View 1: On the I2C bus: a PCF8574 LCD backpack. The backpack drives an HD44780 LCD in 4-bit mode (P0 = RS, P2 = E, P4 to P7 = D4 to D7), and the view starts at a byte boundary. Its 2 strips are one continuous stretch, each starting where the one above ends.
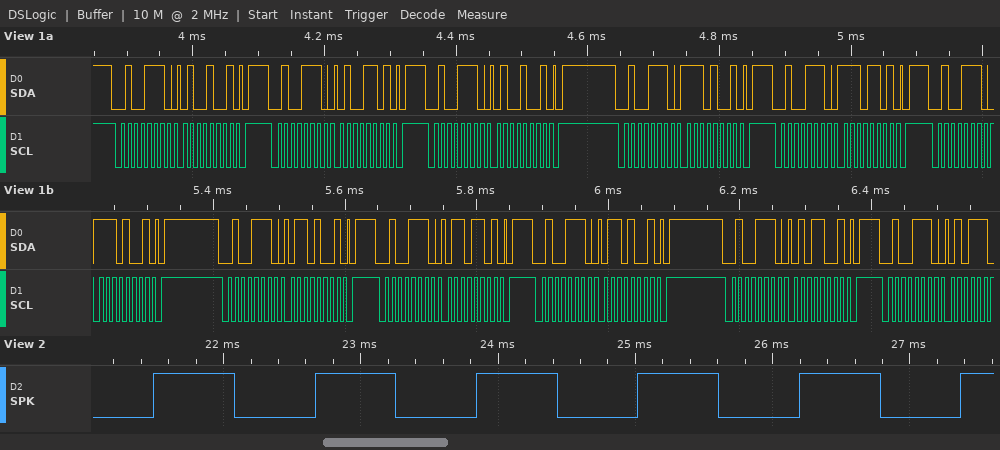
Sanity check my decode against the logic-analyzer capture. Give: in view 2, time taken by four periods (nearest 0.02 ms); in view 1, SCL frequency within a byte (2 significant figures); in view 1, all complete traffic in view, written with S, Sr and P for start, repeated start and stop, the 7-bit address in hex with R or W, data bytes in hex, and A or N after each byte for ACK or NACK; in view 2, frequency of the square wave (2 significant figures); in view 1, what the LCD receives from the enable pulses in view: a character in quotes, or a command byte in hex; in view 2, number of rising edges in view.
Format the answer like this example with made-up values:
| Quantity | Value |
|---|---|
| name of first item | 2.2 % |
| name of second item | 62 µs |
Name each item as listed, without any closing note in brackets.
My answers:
| Quantity | Value |
|---|---|
| in view 2, time taken by four periods | 4.70 ms |
| in view 1, SCL frequency within a byte | 100 kHz |
| in view 1, all complete traffic in view, written with S, Sr and P for start, repeated start and stop, the 7-bit address in hex with R or W, data bytes in hex, and A or N after each byte for ACK or NACK | S 27W A 49 A P S 27W A 4D A P S 27W A 49 A P S 27W A E9 A P S 27W A ED A P S 27W A E9 A P S 27W A 69 A P S 27W A 6D A P S 27W A 69 A P S 27W A 59 A P S 27W A |
| in view 2, frequency of the square wave | 850 Hz |
| in view 1, what the LCD receives from the enable pulses in view: a character in quotes, or a command byte in hex | 'N' |
| in view 2, number of rising edges in view | 6 |
